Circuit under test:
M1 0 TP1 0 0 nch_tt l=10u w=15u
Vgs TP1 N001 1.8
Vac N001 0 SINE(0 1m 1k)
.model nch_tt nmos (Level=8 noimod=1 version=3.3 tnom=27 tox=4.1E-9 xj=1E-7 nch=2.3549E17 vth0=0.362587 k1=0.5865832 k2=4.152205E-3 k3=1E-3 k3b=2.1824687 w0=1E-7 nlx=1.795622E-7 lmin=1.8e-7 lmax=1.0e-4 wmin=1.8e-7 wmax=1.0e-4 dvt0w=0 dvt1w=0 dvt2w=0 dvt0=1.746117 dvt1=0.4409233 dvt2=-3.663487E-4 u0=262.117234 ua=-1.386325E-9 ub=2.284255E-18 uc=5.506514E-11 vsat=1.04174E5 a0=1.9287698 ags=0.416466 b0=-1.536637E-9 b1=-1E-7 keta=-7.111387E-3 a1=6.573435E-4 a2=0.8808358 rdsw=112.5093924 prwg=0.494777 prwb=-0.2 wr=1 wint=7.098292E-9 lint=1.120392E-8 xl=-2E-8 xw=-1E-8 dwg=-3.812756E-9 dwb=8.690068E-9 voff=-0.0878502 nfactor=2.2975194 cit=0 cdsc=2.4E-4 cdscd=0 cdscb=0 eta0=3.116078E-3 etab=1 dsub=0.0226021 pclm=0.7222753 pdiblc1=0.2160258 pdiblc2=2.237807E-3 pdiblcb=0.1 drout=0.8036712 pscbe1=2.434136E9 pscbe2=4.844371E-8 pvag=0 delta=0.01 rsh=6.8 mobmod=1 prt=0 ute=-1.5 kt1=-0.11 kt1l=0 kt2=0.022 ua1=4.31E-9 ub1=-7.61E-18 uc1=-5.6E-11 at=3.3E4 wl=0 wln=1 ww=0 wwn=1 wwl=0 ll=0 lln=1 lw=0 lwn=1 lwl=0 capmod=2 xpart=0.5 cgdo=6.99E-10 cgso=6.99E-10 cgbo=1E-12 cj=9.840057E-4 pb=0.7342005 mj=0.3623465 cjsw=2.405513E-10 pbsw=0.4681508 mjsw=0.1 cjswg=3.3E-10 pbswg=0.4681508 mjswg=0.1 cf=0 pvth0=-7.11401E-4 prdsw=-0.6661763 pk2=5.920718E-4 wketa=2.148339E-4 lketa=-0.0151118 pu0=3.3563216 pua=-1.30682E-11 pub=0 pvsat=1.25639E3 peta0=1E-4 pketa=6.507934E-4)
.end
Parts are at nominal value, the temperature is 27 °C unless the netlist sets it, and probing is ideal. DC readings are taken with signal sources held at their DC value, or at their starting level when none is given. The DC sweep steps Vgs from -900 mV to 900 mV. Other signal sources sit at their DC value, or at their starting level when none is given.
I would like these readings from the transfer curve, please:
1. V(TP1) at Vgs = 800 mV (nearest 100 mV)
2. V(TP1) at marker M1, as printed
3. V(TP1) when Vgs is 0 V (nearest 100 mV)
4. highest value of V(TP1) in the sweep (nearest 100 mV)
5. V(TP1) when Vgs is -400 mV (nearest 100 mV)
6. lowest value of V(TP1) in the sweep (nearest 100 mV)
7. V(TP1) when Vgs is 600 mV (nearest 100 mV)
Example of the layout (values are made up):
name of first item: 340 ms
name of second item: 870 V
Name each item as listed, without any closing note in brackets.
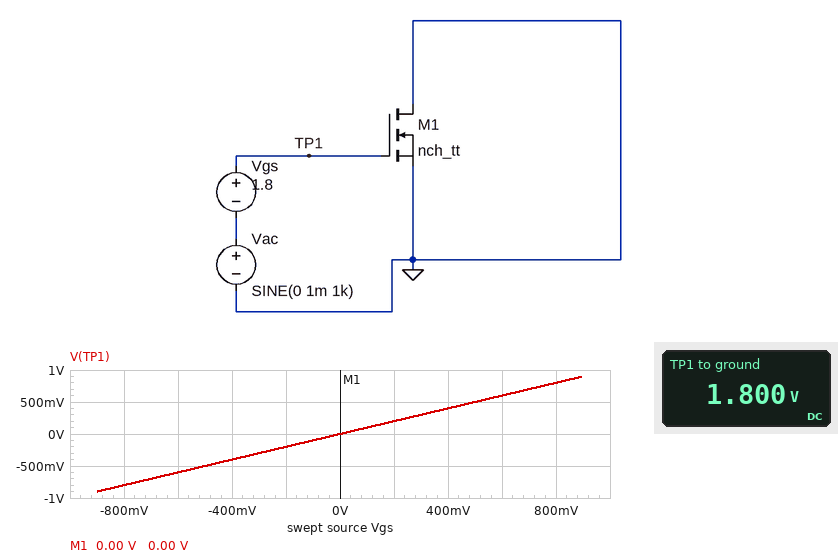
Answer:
V(TP1) at Vgs = 800 mV: 800 mV
V(TP1) at marker M1, as printed: 0.00 V
V(TP1) when Vgs is 0 V: 0 V
highest value of V(TP1) in the sweep: 900 mV
V(TP1) when Vgs is -400 mV: -400 mV
lowest value of V(TP1) in the sweep: -900 mV
V(TP1) when Vgs is 600 mV: 600 mV
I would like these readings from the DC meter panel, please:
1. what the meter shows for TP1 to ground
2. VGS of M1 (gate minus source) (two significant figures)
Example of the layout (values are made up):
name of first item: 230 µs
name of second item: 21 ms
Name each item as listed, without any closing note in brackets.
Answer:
what the meter shows for TP1 to ground: 1.800 V
VGS of M1 (gate minus source): 1.8 V
